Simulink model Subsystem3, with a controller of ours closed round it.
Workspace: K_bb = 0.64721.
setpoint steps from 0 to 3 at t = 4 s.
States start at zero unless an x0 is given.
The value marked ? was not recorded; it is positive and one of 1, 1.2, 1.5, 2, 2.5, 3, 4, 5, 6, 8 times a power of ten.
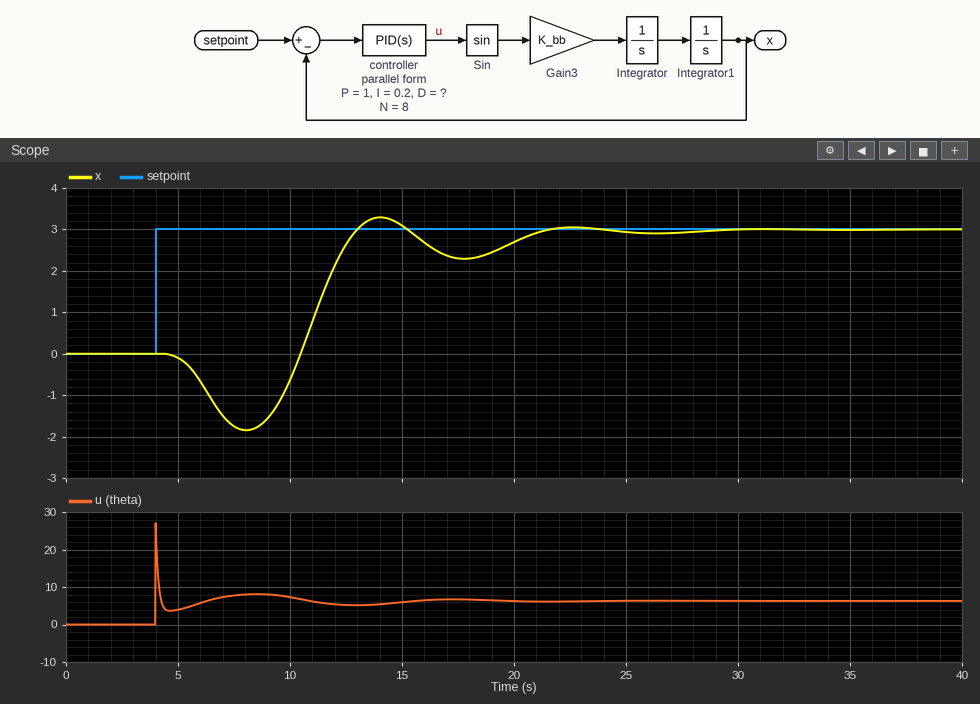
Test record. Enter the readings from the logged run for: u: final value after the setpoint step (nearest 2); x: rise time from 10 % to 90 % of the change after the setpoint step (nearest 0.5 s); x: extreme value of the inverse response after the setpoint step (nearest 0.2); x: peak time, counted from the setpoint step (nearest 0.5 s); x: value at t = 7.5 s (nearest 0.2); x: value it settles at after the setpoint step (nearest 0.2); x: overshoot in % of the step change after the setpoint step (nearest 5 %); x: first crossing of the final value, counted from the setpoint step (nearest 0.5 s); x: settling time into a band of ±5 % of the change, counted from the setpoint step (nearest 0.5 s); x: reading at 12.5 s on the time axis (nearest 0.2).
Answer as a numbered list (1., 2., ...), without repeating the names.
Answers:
1. 6
2. 2.0 s
3. -1.8
4. 10.0 s
5. -1.8
6. 3.0
7. 10 %
8. 9.0 s
9. 16.5 s
10. 2.6
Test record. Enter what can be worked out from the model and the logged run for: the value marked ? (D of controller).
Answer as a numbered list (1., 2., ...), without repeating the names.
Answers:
1. 1
